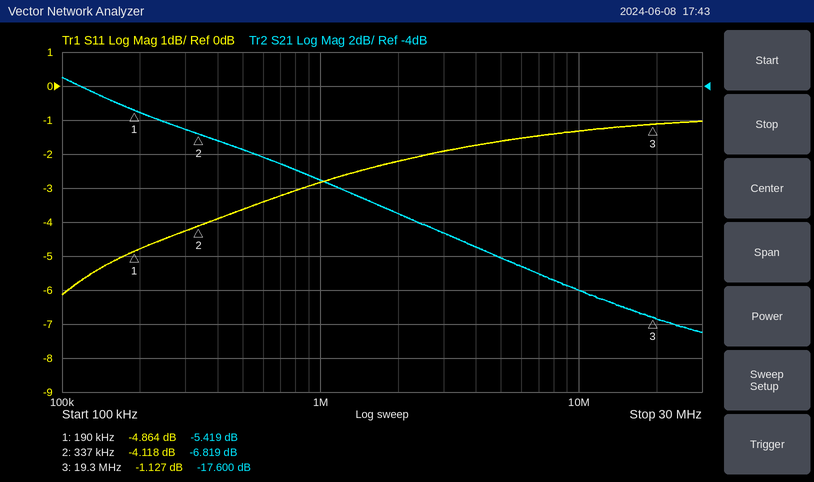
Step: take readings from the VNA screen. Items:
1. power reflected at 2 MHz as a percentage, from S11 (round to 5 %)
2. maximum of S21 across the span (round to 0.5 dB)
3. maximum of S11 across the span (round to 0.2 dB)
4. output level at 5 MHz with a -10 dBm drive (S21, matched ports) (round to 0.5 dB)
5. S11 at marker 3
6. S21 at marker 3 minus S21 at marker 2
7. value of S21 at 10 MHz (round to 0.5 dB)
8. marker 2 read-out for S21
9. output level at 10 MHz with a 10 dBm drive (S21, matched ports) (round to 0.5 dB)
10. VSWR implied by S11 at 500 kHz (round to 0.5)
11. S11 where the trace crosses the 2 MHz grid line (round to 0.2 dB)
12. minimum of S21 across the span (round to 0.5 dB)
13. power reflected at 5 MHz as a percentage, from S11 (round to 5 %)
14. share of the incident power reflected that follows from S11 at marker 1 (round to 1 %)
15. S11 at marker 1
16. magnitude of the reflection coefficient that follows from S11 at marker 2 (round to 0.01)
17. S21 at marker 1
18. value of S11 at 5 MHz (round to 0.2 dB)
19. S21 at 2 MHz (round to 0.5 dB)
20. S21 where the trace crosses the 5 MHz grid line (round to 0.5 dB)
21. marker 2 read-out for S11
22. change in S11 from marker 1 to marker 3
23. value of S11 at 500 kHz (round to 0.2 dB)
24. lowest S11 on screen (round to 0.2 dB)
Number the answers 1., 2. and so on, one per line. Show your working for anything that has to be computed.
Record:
1. 10^(-2.2/10) ≈ 60 %
2. -3.5 dB
3. -1.0 dB
4. -10 dBm + (-14.0 dB) = -24.0 dBm
5. -1.127 dB
6. -17.6 − (-6.819) = -10.781 dB
7. -16.0 dB
8. -6.819 dB
9. 10 dBm + (-16.0 dB) = -6.0 dBm
10. |Γ| = 10^(-3.6/20) = 0.6607; VSWR = (1 + 0.6607)/(1 − 0.6607) ≈ 4.89, so 5.0 to the nearest 0.5
11. -2.2 dB
12. -18.5 dB
13. 10^(-1.6/10) ≈ 69.2 %, so 70 % to the nearest 5 %
14. 10^(-4.864/10) ≈ 33 %
15. -4.864 dB
16. 10^(-4.118/20) ≈ 0.62
17. -5.419 dB
18. -1.6 dB
19. -11.5 dB
20. -14.0 dB
21. -4.118 dB
22. -1.127 − (-4.864) = 3.737 dB
23. -3.6 dB
24. -6.2 dB
